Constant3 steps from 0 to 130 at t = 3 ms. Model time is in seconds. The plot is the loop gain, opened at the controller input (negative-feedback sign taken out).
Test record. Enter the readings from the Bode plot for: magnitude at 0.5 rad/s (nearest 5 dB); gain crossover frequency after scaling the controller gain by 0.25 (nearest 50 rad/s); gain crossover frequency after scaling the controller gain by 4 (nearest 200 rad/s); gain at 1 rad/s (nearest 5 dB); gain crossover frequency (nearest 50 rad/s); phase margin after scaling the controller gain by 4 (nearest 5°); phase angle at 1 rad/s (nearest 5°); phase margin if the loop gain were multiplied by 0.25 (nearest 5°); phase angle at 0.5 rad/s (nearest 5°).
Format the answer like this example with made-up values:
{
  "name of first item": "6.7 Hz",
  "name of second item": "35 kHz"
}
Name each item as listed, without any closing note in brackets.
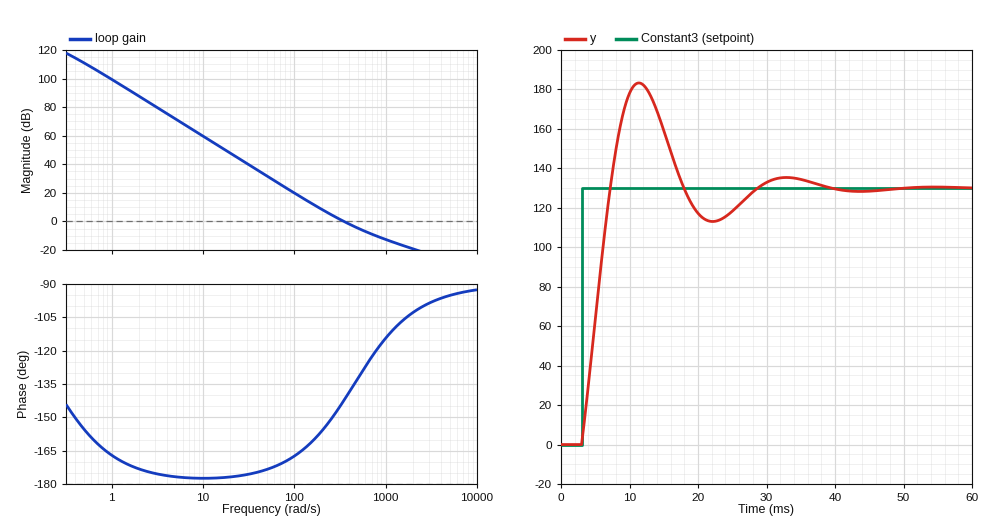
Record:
{
  "magnitude at 0.5 rad/s": "110 dB",
  "gain crossover frequency after scaling the controller gain by 0.25": "150 rad/s",
  "gain crossover frequency after scaling the controller gain by 4": "1000 rad/s",
  "gain at 1 rad/s": "100 dB",
  "gain crossover frequency": "350 rad/s",
  "phase margin after scaling the controller gain by 4": "65°",
  "phase angle at 1 rad/s": "-165°",
  "phase margin if the loop gain were multiplied by 0.25": "20°",
  "phase angle at 0.5 rad/s": "-155°"
}
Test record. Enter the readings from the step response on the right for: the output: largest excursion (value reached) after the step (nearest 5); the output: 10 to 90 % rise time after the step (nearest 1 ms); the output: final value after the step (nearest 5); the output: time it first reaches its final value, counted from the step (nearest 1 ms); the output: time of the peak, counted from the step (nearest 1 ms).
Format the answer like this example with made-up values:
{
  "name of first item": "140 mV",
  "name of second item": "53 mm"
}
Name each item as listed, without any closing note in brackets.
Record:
{
  "the output: largest excursion (value reached) after the step": "185",
  "the output: 10 to 90 % rise time after the step": "3 ms",
  "the output: final value after the step": "130",
  "the output: time it first reaches its final value, counted from the step": "4 ms",
  "the output: time of the peak, counted from the step": "8 ms"
}
